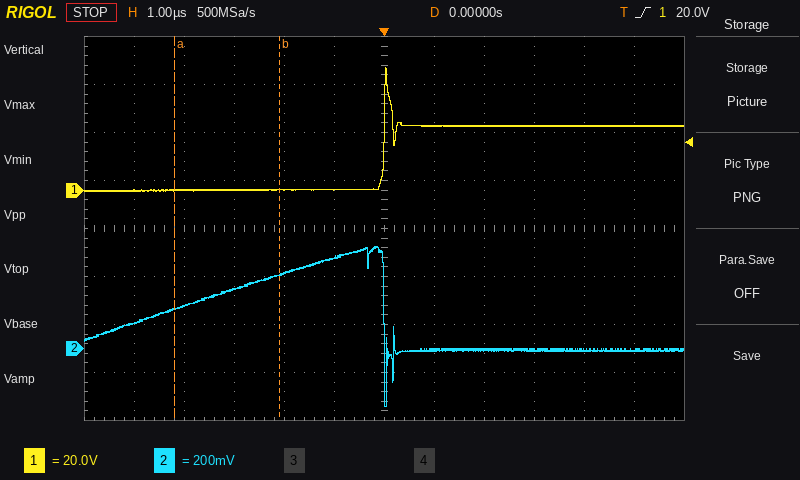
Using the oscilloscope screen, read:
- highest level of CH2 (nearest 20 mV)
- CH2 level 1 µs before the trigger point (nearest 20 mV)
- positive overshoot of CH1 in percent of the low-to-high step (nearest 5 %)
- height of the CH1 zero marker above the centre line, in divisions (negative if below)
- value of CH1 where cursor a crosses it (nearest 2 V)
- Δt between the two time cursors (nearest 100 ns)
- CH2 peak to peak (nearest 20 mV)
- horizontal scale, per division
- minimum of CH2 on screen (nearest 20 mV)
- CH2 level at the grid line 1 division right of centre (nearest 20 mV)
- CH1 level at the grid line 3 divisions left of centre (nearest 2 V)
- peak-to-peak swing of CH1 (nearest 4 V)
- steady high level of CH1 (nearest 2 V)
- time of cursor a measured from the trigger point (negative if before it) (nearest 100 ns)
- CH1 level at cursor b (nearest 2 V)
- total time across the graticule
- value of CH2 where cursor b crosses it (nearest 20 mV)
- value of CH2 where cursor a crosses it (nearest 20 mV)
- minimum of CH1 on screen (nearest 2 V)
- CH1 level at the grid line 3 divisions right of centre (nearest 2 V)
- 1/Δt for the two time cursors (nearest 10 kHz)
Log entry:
420 mV
380 mV
90 %
+0.8 div
0 V
2.1 µs
660 mV
1 µs
-240 mV
0 mV
0 V
52 V
26 V
-4.2 µs
0 V
12 µs
300 mV
160 mV
0 V
26 V
480 kHz
